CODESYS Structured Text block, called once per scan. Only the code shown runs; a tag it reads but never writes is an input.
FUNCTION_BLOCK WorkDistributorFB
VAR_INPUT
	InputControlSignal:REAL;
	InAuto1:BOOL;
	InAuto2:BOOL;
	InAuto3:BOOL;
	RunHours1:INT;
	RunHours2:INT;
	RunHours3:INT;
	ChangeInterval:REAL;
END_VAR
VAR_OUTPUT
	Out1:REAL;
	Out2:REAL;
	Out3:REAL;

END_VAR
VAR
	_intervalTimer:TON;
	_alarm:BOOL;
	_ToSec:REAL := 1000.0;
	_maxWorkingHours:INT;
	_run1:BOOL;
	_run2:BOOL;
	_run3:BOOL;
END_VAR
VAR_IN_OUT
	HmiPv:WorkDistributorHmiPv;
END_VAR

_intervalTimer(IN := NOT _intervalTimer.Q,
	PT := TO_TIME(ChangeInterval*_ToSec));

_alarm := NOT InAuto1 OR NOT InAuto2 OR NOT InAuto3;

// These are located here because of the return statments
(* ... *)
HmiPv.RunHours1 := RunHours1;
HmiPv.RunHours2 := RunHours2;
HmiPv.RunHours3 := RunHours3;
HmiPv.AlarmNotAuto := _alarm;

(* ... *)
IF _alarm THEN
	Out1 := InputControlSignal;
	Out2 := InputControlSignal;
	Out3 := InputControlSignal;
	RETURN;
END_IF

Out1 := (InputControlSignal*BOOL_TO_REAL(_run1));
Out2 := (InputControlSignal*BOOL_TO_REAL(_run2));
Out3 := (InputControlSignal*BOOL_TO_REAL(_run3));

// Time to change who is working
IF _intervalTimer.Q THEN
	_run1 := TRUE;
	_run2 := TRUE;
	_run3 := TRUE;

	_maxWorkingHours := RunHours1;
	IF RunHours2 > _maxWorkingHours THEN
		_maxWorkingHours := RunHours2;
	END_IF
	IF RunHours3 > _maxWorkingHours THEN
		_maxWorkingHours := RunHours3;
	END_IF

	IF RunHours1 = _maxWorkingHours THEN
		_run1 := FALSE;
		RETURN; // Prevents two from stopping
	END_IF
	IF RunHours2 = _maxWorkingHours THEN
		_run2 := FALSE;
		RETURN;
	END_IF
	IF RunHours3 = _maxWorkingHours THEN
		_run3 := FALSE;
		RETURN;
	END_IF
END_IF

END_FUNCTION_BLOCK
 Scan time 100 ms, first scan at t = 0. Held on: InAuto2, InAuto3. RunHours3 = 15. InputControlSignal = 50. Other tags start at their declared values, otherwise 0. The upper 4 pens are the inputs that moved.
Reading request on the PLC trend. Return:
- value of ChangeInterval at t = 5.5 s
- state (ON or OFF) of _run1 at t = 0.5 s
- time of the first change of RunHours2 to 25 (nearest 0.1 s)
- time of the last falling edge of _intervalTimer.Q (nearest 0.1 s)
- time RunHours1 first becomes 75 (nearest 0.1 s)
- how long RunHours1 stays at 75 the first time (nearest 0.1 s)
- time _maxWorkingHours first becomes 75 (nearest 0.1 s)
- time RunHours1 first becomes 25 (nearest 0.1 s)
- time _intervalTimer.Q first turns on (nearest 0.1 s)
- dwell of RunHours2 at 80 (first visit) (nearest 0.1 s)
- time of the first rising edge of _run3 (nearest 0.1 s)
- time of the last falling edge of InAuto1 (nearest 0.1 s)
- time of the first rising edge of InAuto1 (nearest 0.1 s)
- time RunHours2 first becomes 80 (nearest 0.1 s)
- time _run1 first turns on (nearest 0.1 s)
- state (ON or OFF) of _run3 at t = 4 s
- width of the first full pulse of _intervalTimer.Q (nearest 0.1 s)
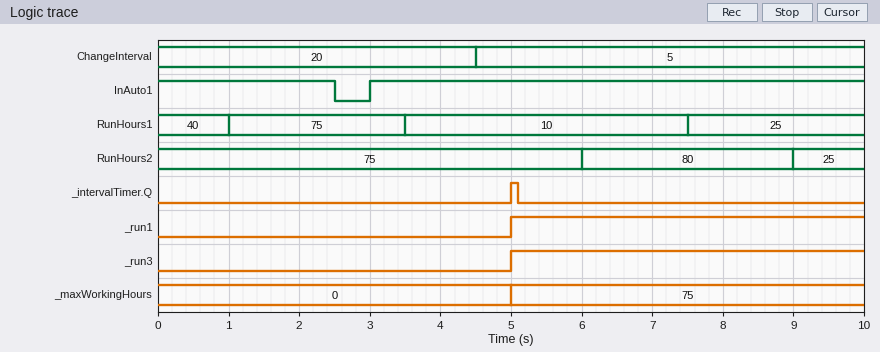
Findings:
5
OFF
9.0 s
5.1 s
1.0 s
2.5 s
5.0 s
7.5 s
5.0 s
3.0 s
5.0 s
2.5 s
3.0 s
6.0 s
5.0 s
OFF
0.1 s
